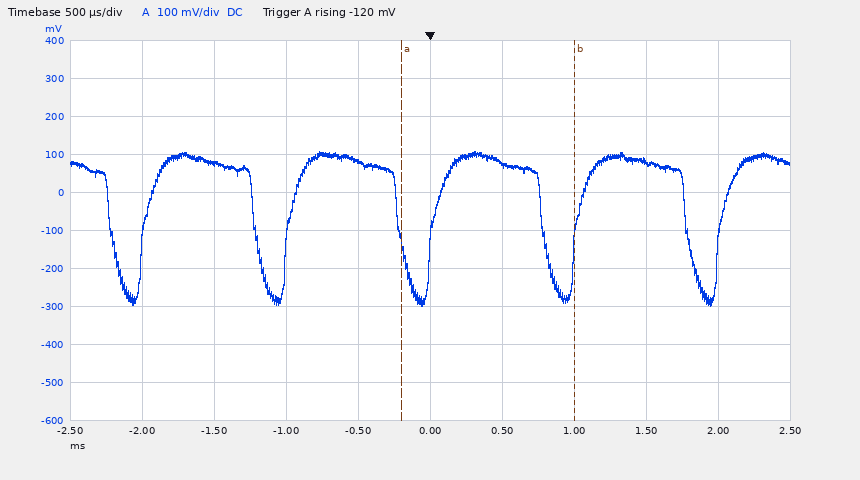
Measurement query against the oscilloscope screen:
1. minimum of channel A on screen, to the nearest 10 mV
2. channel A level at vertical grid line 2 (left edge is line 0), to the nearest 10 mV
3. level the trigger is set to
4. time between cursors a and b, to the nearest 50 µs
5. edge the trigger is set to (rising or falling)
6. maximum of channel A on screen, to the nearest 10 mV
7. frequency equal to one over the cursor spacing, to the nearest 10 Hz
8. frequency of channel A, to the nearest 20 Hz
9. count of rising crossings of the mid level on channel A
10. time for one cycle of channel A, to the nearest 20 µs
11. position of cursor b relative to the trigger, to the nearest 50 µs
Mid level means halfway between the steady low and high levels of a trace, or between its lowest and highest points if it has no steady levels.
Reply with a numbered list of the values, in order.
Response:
1. -300 mV
2. 80 mV
3. -120 mV
4. 1.20 ms
5. rising
6. 110 mV
7. 830 Hz
8. 1.00 kHz
9. 5
10. 1.00 ms
11. +1.00 ms
